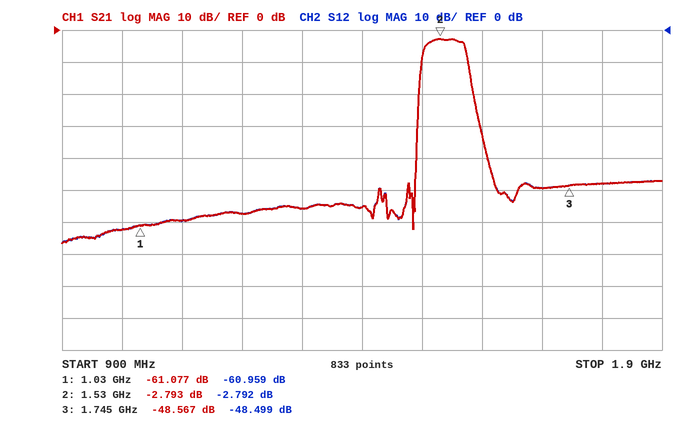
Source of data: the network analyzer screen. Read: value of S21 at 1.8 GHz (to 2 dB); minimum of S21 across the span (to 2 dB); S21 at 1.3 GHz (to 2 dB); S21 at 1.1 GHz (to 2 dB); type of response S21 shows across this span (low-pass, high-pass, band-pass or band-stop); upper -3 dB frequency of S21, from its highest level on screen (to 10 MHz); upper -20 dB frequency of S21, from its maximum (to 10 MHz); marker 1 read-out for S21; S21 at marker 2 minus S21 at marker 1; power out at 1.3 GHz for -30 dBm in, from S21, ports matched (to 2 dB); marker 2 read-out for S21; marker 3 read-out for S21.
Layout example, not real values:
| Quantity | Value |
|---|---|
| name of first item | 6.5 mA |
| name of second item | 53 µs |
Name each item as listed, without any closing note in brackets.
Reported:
| Quantity | Value |
|---|---|
| value of S21 at 1.8 GHz | -48 dB |
| minimum of S21 across the span | -66 dB |
| S21 at 1.3 GHz | -56 dB |
| S21 at 1.1 GHz | -60 dB |
| type of response S21 shows across this span | band-pass |
| upper -3 dB frequency of S21, from its highest level on screen | 1.57 GHz |
| upper -20 dB frequency of S21, from its maximum | 1.59 GHz |
| marker 1 read-out for S21 | -61.077 dB |
| S21 at marker 2 minus S21 at marker 1 | 58.284 dB |
| power out at 1.3 GHz for -30 dBm in, from S21, ports matched | -86 dBm |
| marker 2 read-out for S21 | -2.793 dB |
| marker 3 read-out for S21 | -48.567 dB |
